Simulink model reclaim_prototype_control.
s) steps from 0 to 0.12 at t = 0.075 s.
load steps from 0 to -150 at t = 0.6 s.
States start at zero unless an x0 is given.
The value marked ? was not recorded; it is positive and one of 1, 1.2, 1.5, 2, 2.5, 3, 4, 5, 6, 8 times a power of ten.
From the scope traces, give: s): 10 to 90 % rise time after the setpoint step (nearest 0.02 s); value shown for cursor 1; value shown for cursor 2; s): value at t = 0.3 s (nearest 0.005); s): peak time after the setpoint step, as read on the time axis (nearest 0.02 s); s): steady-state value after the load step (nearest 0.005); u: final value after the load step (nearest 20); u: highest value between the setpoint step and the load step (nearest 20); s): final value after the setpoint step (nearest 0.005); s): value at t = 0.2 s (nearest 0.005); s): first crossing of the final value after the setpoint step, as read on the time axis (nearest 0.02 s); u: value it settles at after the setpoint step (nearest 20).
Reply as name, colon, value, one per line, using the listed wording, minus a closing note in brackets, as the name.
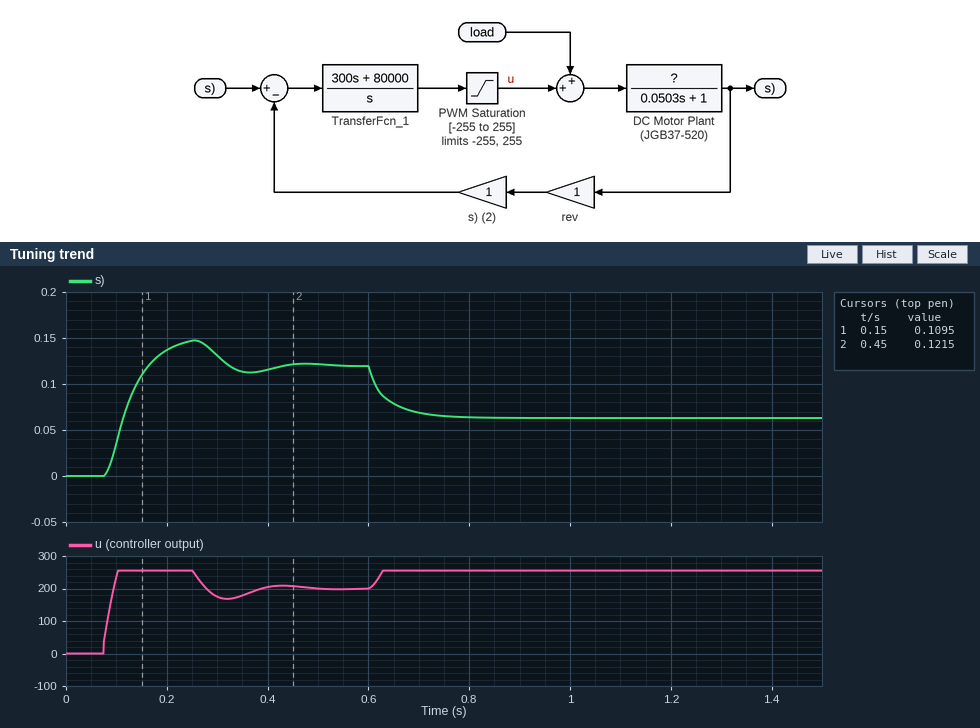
s): 10 to 90 % rise time after the setpoint step: 0.06 s
value shown for cursor 1: 0.1095
value shown for cursor 2: 0.1215
s): value at t = 0.3 s: 0.130
s): peak time after the setpoint step, as read on the time axis: 0.26 s
s): steady-state value after the load step: 0.065
u: final value after the load step: 260
u: highest value between the setpoint step and the load step: 260
s): final value after the setpoint step: 0.120
s): value at t = 0.2 s: 0.135
s): first crossing of the final value after the setpoint step, as read on the time axis: 0.16 s
u: value it settles at after the setpoint step: 200
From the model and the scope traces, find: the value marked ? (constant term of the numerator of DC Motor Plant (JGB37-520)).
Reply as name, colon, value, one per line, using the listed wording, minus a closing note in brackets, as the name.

the value marked ? (constant term of the numerator of DC Motor Plant (JGB37-520)): 0.0006
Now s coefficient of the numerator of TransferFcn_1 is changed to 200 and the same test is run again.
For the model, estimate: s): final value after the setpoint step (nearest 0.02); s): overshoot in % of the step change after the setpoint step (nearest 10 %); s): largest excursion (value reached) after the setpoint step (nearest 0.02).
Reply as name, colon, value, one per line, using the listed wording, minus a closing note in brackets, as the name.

s): final value after the setpoint step: 0.12
s): overshoot in % of the step change after the setpoint step: 20 %
s): largest excursion (value reached) after the setpoint step: 0.14
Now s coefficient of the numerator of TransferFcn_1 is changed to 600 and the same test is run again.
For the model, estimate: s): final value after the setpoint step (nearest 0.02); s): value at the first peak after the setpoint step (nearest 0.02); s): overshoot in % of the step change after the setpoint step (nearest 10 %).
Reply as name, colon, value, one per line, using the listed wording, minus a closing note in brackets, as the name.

s): final value after the setpoint step: 0.12
s): value at the first peak after the setpoint step: 0.14
s): overshoot in % of the step change after the setpoint step: 20 %
